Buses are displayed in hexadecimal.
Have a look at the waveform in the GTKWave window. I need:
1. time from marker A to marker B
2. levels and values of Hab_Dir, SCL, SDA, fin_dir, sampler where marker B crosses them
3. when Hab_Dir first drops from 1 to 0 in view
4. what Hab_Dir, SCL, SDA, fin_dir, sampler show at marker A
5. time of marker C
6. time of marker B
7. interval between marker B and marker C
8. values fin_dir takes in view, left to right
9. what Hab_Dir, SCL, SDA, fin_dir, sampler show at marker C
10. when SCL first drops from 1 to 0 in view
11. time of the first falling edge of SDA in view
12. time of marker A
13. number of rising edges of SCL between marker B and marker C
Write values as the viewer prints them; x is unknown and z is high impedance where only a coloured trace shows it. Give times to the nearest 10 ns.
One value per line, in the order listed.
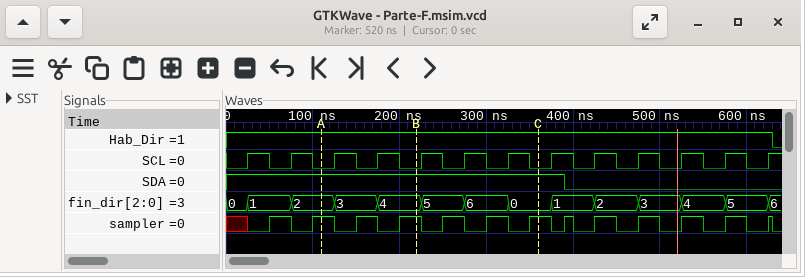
110 ns
Hab_Dir=1, SCL=0, SDA=1, fin_dir=4, sampler=1
630 ns
Hab_Dir=1, SCL=0, SDA=1, fin_dir=2, sampler=1
360 ns
220 ns
140 ns
0, 1, 2, 3, 4, 5, 6, 0, 1, 2, 3, 4, 5, 6
Hab_Dir=1, SCL=0, SDA=1, fin_dir=0, sampler=1
50 ns
390 ns
110 ns
3
